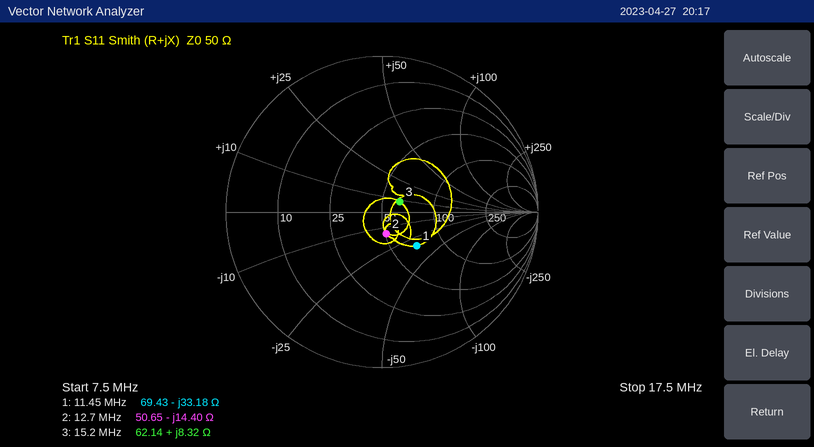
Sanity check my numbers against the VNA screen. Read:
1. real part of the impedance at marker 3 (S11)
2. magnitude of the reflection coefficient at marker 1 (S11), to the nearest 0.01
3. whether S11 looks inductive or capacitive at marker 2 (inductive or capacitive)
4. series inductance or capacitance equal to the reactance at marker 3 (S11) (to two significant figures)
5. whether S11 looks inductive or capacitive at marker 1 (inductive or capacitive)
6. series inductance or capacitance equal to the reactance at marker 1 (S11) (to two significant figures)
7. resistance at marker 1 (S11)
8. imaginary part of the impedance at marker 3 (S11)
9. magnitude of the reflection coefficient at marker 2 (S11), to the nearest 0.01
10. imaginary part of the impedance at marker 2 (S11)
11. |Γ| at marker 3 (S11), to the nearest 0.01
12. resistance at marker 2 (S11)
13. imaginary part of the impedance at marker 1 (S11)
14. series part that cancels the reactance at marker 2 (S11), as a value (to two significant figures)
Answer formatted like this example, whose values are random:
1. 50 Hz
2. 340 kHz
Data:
1. 62.14 Ω
2. 0.31
3. capacitive
4. 87 nH
5. capacitive
6. 420 pF
7. 69.43 Ω
8. +8.32 Ω
9. 0.14
10. -14.40 Ω
11. 0.13
12. 50.65 Ω
13. -33.18 Ω
14. 180 nH
